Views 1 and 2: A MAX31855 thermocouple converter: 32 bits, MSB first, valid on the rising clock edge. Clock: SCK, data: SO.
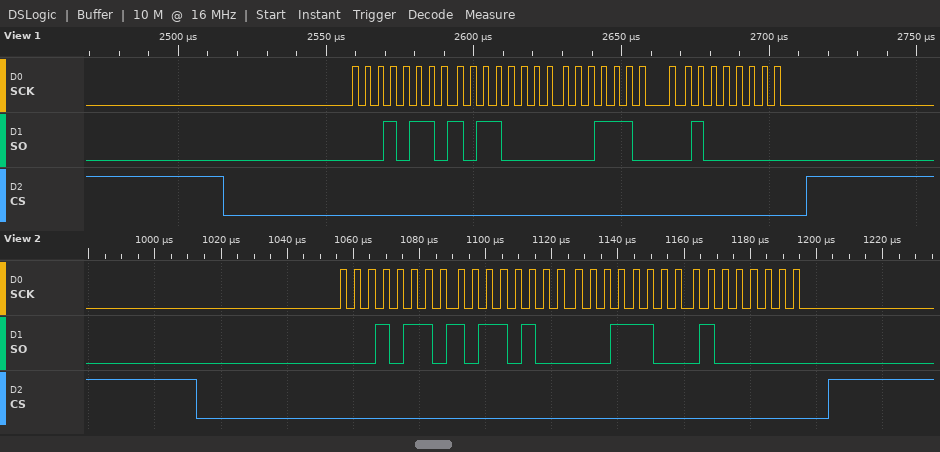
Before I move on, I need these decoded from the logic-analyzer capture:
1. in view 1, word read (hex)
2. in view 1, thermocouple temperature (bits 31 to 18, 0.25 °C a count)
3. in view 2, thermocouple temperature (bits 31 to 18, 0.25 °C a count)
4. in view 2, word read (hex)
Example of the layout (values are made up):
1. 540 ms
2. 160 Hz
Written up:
1. 0x16B01C40
2. 363.00 °C
3. 363.25 °C
4. 0x16B41C40
